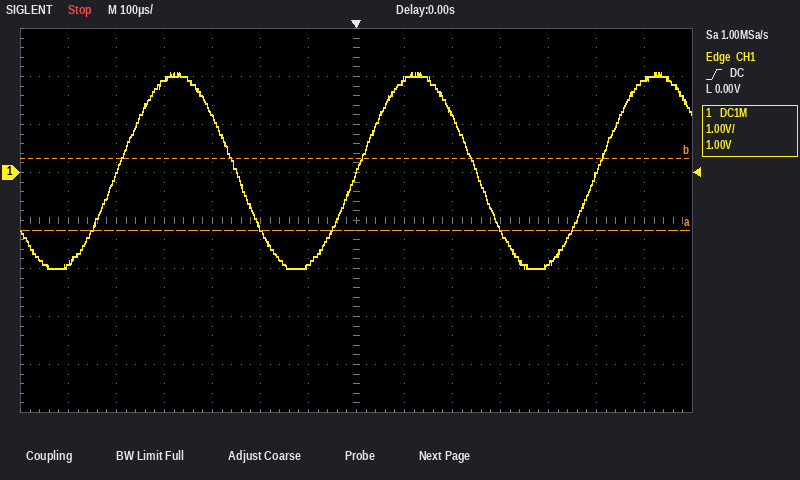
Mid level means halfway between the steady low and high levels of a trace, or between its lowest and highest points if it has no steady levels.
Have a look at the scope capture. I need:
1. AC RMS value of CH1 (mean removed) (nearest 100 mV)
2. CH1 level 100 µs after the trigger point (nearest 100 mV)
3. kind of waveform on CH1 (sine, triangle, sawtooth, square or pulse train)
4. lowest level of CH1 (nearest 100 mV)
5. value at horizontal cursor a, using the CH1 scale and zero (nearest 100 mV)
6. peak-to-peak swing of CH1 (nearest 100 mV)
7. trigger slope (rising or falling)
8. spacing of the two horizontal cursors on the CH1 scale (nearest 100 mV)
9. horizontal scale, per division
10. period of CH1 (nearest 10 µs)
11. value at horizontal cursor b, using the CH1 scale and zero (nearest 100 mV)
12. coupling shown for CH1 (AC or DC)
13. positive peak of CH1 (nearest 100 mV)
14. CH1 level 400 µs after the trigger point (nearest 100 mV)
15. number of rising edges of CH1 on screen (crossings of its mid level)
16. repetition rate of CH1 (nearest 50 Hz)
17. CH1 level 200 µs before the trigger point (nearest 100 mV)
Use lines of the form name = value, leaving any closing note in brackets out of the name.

AC RMS value of CH1 (mean removed) = 1.4 V
CH1 level 100 µs after the trigger point = 1.9 V
kind of waveform on CH1 = sine
lowest level of CH1 = -2.0 V
value at horizontal cursor a, using the CH1 scale and zero = -1.2 V
peak-to-peak swing of CH1 = 4.1 V
trigger slope = rising
spacing of the two horizontal cursors on the CH1 scale = 1.5 V
horizontal scale, per division = 100 µs
period of CH1 = 500 µs
value at horizontal cursor b, using the CH1 scale and zero = 300 mV
coupling shown for CH1 = DC
positive peak of CH1 = 2.1 V
CH1 level 400 µs after the trigger point = -1.9 V
number of rising edges of CH1 on screen = 3
repetition rate of CH1 = 2.00 kHz
CH1 level 200 µs before the trigger point = -1.1 V
